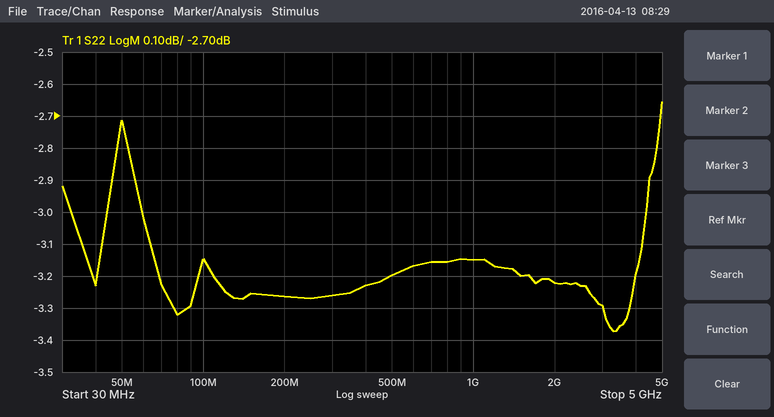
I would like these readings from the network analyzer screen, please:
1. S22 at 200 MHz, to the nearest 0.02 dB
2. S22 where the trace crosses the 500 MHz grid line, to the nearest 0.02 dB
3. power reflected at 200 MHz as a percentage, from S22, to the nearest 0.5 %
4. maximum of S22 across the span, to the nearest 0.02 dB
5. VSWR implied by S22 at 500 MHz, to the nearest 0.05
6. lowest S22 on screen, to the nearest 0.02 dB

-3.26 dB
-3.20 dB
47.0 %
-2.66 dB
5.50
-3.38 dB
